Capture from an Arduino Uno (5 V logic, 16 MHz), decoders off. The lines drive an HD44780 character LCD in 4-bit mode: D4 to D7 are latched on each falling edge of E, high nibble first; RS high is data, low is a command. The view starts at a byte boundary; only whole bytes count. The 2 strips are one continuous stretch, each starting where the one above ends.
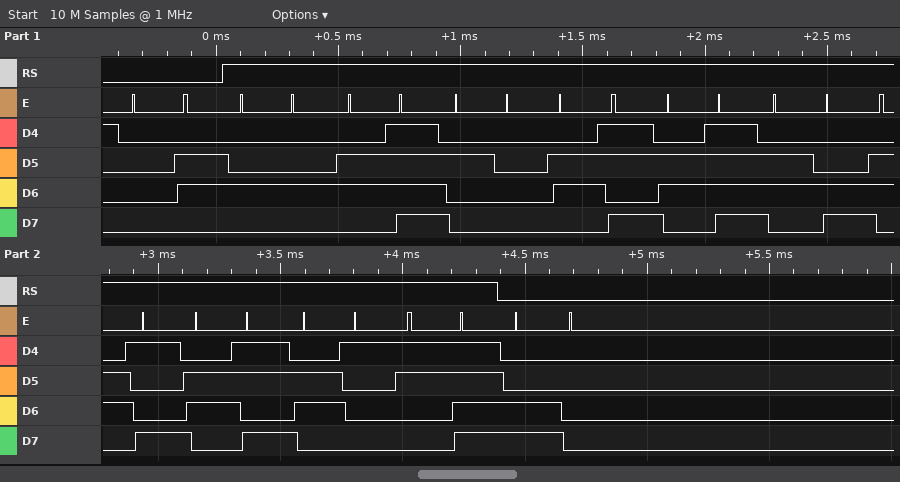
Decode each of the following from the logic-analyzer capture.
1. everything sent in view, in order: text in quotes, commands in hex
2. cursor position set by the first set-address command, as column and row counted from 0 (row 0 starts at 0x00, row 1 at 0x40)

0x06 "Do kolika?" 0xC0
column 0, row 1
